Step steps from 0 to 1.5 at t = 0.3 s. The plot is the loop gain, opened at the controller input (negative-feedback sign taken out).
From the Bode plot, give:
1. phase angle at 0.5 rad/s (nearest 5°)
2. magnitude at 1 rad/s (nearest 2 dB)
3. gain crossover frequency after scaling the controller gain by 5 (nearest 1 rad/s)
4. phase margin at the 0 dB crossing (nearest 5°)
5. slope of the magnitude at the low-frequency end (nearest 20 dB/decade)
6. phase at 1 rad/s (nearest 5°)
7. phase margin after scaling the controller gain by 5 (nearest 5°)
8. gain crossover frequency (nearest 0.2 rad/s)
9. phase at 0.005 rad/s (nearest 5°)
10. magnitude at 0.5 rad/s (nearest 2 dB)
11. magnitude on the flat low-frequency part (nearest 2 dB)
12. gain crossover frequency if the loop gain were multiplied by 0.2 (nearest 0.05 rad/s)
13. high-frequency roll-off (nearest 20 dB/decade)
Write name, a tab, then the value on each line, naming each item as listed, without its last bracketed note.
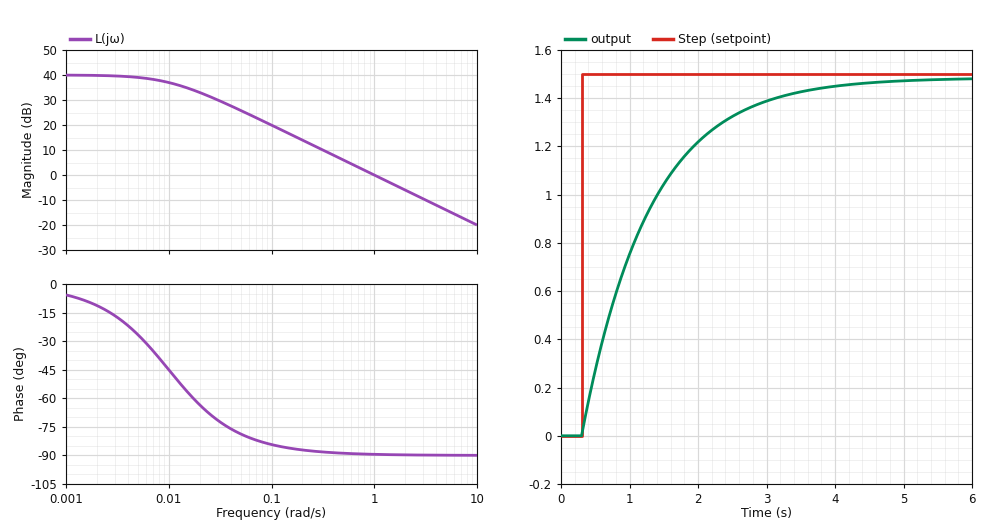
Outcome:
phase angle at 0.5 rad/s	-90°
magnitude at 1 rad/s	0 dB
gain crossover frequency after scaling the controller gain by 5	5 rad/s
phase margin at the 0 dB crossing	90°
slope of the magnitude at the low-frequency end	0 dB/decade
phase at 1 rad/s	-90°
phase margin after scaling the controller gain by 5	90°
gain crossover frequency	1.0 rad/s
phase at 0.005 rad/s	-25°
magnitude at 0.5 rad/s	6 dB
magnitude on the flat low-frequency part	40 dB
gain crossover frequency if the loop gain were multiplied by 0.2	0.20 rad/s
high-frequency roll-off	-20 dB/decade
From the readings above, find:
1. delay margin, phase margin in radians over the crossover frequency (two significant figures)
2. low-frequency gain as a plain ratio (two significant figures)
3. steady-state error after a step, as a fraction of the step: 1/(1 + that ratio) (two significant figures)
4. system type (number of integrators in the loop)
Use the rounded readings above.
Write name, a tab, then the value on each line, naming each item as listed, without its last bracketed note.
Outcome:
delay margin, phase margin in radians over the crossover frequency	1.6 s
low-frequency gain as a plain ratio	100
steady-state error after a step, as a fraction of the step: 1/(1 + that ratio)	0.0099
system type	0
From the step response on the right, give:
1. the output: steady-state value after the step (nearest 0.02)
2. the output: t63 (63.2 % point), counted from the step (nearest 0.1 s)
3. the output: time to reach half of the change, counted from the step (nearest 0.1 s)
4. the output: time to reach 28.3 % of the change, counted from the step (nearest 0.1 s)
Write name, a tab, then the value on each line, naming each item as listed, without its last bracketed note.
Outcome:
the output: steady-state value after the step	1.48
the output: t63 (63.2 % point), counted from the step	1.0 s
the output: time to reach half of the change, counted from the step	0.7 s
the output: time to reach 28.3 % of the change, counted from the step	0.3 s
